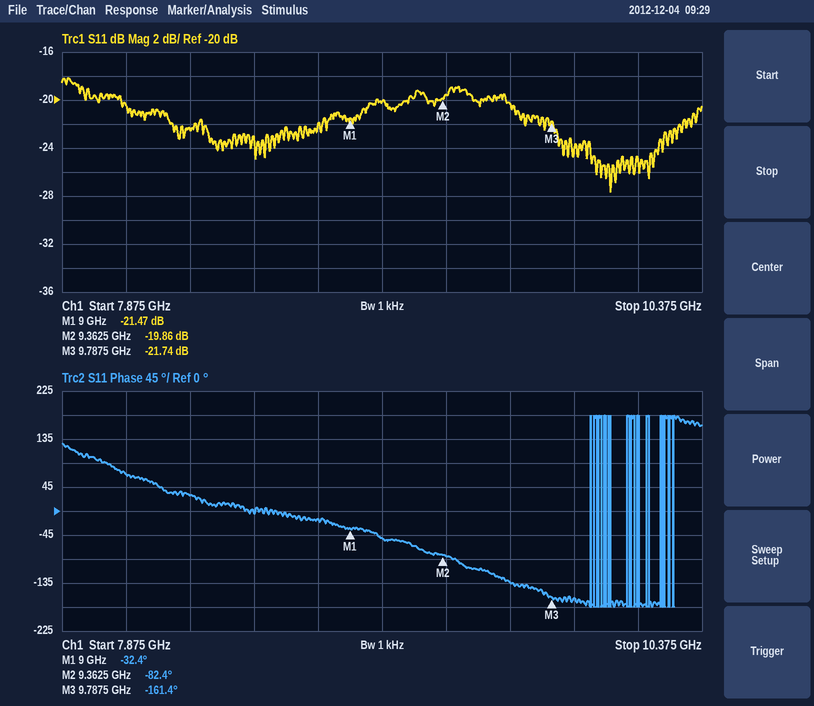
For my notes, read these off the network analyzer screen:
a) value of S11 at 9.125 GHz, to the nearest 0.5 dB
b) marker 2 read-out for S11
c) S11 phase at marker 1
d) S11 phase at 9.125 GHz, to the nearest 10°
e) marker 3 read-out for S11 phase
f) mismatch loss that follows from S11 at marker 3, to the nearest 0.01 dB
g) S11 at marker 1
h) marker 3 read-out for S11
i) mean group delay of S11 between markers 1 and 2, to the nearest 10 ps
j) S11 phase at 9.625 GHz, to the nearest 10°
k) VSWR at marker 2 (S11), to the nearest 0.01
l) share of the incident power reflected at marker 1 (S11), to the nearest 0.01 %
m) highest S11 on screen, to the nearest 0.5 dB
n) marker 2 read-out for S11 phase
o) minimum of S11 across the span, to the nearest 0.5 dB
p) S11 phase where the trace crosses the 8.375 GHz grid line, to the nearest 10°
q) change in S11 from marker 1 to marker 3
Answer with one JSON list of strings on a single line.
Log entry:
["-20.0 dB", "-19.86 dB", "-32.4°", "-50°", "-161.4°", "0.03 dB", "-21.47 dB", "-21.74 dB", "380 ps", "-130°", "1.23", "0.71 %", "-18.0 dB", "-82.4°", "-27.5 dB", "30°", "-0.27 dB"]
